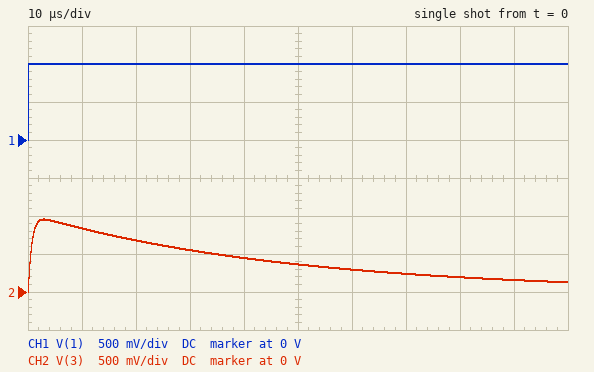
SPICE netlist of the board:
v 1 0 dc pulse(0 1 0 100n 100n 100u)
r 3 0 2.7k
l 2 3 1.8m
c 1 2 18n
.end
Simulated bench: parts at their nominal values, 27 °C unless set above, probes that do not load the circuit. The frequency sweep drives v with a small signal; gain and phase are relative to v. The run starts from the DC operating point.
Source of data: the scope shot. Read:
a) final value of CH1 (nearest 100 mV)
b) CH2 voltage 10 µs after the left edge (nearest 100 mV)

1.0 V
800 mV
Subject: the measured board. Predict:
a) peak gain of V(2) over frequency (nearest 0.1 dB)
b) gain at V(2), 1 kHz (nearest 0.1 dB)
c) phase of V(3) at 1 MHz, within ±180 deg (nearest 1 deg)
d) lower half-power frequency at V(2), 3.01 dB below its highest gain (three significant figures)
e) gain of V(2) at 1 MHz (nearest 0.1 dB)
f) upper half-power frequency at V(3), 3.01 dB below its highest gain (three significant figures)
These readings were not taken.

0.1 dB
-10.7 dB
-77 deg
3.31 kHz
0 dB
242 kHz
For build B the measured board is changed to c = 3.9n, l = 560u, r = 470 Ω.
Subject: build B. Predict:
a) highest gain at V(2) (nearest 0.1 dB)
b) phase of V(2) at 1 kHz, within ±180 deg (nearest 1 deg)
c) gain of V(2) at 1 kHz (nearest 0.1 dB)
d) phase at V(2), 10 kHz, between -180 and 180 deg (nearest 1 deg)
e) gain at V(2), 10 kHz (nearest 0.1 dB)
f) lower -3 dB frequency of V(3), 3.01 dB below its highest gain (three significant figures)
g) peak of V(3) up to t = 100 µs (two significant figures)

2.5 dB
90 deg
-38.8 dB
88 deg
-18.7 dB
59.9 kHz
610 mV
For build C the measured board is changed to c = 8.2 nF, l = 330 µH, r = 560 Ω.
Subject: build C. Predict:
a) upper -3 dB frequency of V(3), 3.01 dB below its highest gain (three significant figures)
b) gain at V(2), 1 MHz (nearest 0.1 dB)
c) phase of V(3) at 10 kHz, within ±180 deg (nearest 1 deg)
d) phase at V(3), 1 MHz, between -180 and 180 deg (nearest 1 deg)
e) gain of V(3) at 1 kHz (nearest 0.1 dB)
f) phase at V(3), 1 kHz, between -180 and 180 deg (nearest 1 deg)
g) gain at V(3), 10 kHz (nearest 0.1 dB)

301 kHz
0.1 dB
74 deg
-75 deg
-30.8 dB
88 deg
-11.1 dB
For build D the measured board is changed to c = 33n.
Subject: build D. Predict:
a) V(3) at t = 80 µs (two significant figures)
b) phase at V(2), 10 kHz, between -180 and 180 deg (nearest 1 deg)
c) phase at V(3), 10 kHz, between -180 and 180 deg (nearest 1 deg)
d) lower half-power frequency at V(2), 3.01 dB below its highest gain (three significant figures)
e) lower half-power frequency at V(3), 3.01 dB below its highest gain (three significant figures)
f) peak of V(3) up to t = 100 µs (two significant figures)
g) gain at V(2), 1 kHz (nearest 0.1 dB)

410 mV
10 deg
8 deg
1.80 kHz
1.77 kHz
970 mV
-6.2 dB
